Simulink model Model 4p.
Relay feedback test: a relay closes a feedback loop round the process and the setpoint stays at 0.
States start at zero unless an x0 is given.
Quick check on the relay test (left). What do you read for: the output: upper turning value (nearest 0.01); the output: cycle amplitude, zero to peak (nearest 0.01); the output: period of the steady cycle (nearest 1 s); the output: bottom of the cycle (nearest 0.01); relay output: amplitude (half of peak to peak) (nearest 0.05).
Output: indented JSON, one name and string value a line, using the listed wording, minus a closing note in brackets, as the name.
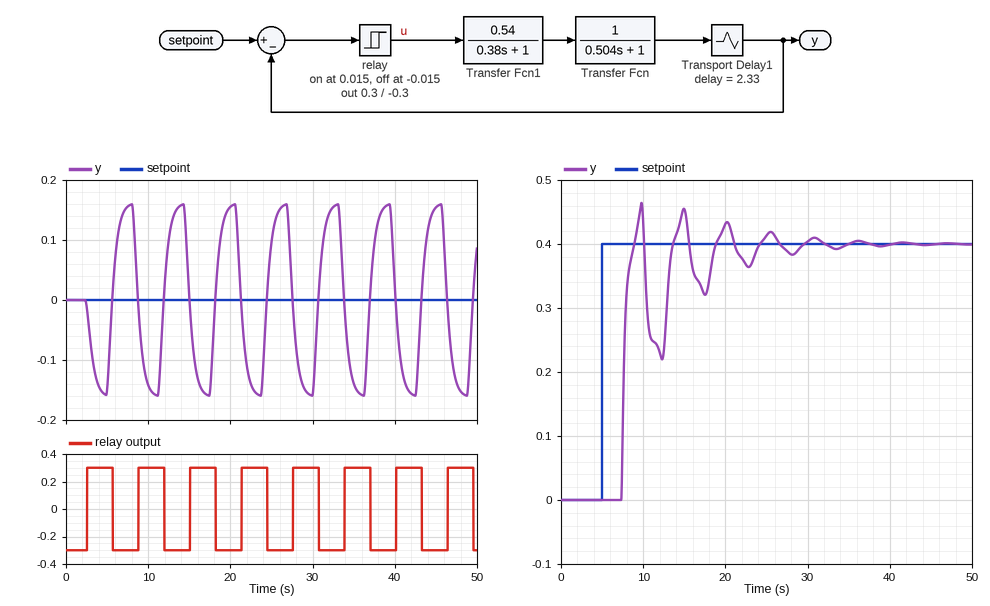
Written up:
{
  "the output: upper turning value": "0.16",
  "the output: cycle amplitude, zero to peak": "0.16",
  "the output: period of the steady cycle": "6 s",
  "the output: bottom of the cycle": "-0.16",
  "relay output: amplitude (half of peak to peak)": "0.30"
}
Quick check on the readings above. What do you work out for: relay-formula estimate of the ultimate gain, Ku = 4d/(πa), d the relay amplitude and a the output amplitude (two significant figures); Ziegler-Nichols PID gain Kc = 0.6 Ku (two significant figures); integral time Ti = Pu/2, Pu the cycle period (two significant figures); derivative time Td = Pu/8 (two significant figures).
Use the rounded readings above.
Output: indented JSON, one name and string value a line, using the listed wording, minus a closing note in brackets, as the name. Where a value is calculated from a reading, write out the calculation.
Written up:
{
  "relay-formula estimate of the ultimate gain, Ku = 4d/(πa), d the relay amplitude and a the output amplitude": "4 × 0.3 / (π × 0.16) = 2.4",
  "Ziegler-Nichols PID gain Kc = 0.6 Ku": "0.6 × 2.4 = 1.4",
  "integral time Ti = Pu/2, Pu the cycle period": "6 / 2 = 3.0 s",
  "derivative time Td = Pu/8": "6 / 8 = 0.75 s"
}
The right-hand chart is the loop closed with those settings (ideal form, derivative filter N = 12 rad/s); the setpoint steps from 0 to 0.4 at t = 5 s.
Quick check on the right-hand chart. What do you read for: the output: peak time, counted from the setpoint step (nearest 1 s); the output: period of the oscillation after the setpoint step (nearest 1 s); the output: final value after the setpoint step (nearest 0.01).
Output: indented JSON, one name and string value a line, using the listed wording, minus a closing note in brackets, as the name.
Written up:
{
  "the output: peak time, counted from the setpoint step": "5 s",
  "the output: period of the oscillation after the setpoint step": "5 s",
  "the output: final value after the setpoint step": "0.40"
}
